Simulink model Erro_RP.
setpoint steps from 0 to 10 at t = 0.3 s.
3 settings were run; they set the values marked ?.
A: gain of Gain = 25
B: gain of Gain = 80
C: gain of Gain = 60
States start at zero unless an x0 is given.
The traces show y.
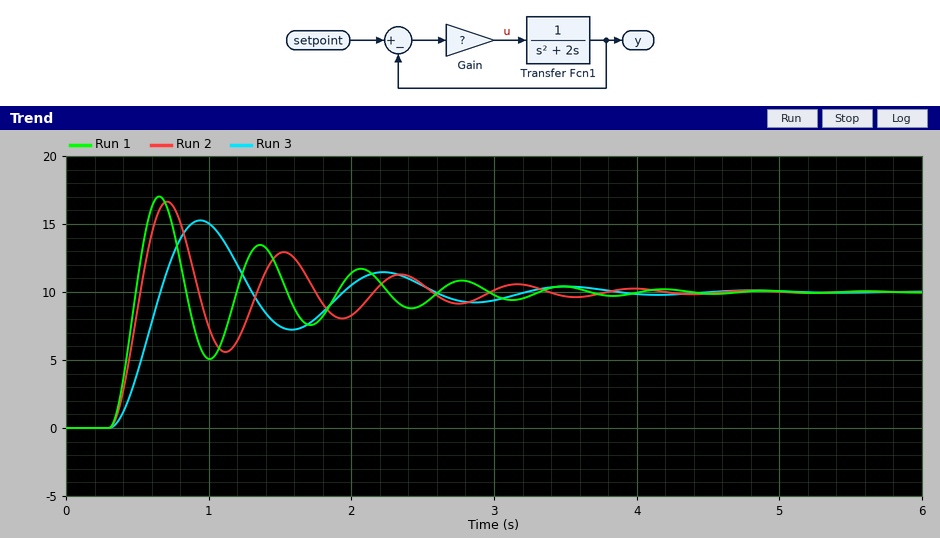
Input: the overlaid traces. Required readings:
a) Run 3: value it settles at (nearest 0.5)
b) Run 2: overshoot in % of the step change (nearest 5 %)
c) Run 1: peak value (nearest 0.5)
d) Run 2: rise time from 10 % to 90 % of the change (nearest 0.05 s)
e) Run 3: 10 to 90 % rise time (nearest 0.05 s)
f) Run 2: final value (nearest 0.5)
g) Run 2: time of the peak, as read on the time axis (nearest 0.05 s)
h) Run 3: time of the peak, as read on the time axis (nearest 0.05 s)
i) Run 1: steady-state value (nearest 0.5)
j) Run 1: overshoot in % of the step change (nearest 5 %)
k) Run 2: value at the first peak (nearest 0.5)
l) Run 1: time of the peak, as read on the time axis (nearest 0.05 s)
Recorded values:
10.0
65 %
17.0
0.15 s
0.25 s
10.0
0.70 s
0.95 s
10.0
70 %
16.5
0.65 s
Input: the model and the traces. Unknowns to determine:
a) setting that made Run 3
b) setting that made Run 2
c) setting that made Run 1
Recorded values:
A
C
B
